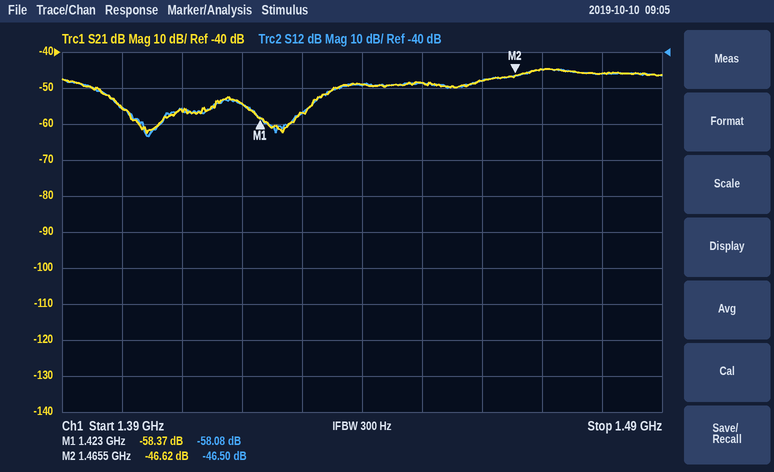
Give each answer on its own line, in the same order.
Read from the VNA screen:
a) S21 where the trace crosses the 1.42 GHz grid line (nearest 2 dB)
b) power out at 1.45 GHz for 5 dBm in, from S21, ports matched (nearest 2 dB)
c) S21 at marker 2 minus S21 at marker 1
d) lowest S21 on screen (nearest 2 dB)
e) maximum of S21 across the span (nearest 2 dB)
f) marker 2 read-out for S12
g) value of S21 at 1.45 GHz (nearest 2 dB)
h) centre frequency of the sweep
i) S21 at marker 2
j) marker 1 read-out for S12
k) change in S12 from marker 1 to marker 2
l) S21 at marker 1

-54 dB
-44 dBm
11.75 dB
-62 dB
-44 dB
-46.50 dB
-48 dB
1.44 GHz
-46.62 dB
-58.08 dB
11.58 dB
-58.37 dB
